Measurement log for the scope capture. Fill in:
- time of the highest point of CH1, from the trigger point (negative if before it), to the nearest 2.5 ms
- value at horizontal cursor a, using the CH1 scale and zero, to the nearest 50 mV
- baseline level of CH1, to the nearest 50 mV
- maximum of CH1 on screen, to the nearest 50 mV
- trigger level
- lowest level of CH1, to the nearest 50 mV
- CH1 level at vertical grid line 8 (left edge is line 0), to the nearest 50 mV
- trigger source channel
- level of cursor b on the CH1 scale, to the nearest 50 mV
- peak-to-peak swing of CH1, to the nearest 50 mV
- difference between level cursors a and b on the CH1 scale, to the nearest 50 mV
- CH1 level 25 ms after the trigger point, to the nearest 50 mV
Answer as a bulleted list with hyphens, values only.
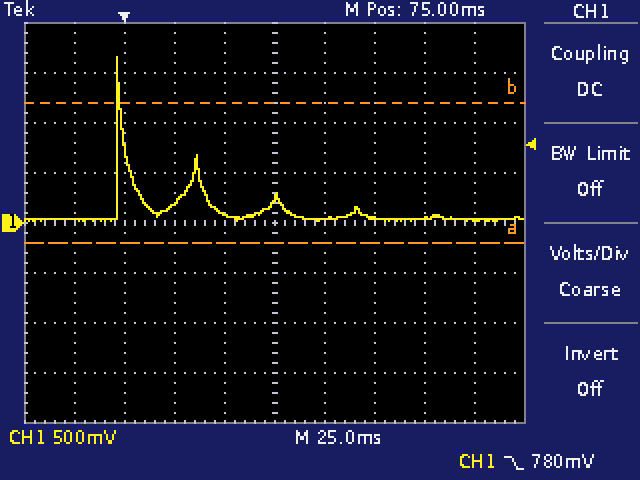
- -2.5 ms
- -200 mV
- 50 mV
- 1.65 V
- 780 mV
- 0 mV
- 50 mV
- CH1
- 1.20 V
- 1.65 V
- 1.40 V
- 200 mV
